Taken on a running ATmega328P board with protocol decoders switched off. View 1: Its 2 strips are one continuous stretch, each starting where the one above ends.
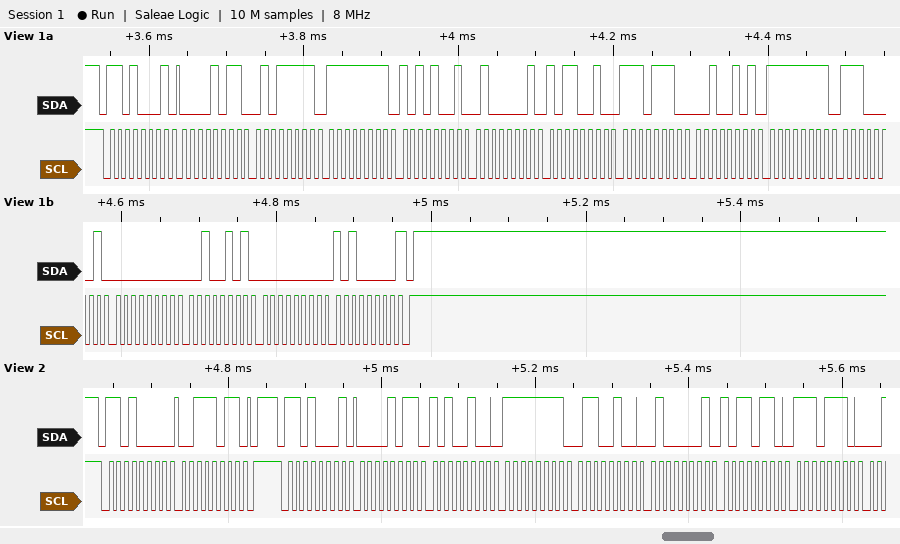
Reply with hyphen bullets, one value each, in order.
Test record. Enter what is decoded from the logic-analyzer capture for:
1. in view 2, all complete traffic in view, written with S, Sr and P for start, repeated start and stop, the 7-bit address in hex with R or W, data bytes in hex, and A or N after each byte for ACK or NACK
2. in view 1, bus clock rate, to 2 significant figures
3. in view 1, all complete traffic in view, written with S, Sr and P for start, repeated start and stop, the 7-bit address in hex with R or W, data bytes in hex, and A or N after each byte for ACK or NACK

- S 68W A 3B A P S 68R A 0B A A4 A FF A 64 A 41 A B6 A EE A
- 100 kHz
- S 68R A 0B A 5F A FF A A9 A 41 A B2 A EE A 25 A FF A E1 A 00 A 25 A 00 A A0 N P
